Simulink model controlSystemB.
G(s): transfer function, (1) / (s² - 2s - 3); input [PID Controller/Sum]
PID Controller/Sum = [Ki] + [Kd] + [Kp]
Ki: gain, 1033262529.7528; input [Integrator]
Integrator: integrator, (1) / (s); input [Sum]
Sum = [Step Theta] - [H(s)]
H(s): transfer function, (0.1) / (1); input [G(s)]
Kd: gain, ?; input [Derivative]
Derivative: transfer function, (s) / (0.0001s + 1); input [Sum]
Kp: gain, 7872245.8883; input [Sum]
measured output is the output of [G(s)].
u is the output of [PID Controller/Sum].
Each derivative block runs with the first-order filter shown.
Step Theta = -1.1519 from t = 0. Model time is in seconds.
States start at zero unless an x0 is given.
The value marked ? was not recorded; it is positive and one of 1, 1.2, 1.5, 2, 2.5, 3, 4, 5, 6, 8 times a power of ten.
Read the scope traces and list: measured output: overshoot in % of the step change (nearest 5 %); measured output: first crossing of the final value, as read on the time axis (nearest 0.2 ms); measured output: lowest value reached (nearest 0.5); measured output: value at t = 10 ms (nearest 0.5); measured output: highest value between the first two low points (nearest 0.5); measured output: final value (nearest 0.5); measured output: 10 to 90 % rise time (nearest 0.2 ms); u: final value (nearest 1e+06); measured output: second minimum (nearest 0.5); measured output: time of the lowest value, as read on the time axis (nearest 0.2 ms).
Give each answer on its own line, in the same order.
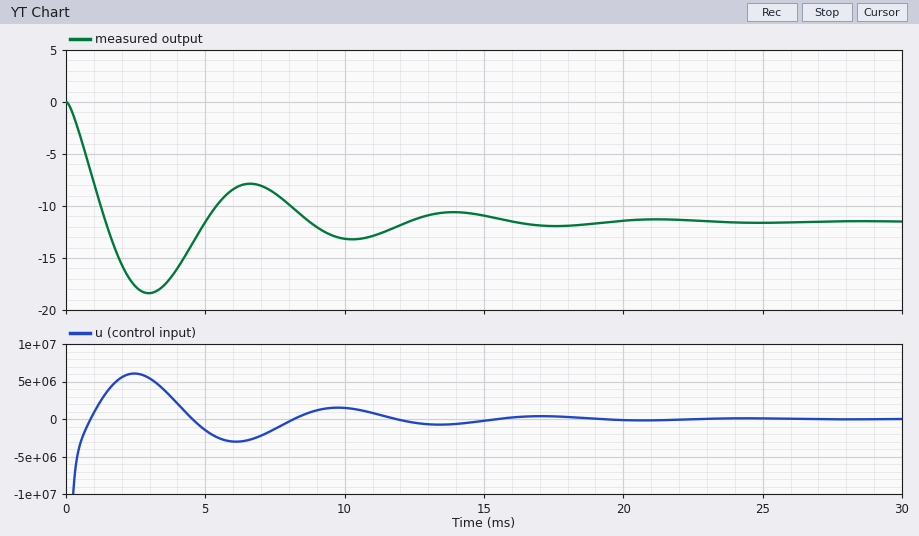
60 %
1.4 ms
-18.5
-13.0
-8.0
-11.5
1.0 ms
0
-13.0
3.0 ms
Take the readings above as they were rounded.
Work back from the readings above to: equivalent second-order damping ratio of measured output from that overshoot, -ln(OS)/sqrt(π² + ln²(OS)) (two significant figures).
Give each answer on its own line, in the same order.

0.16
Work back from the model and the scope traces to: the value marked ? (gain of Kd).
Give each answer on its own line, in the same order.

5000
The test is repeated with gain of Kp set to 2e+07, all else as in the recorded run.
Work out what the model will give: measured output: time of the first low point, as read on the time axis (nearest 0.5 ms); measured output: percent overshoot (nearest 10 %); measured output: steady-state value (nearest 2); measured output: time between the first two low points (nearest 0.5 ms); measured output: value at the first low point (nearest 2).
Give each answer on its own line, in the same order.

2.0 ms
70 %
-12
4.5 ms
-20
